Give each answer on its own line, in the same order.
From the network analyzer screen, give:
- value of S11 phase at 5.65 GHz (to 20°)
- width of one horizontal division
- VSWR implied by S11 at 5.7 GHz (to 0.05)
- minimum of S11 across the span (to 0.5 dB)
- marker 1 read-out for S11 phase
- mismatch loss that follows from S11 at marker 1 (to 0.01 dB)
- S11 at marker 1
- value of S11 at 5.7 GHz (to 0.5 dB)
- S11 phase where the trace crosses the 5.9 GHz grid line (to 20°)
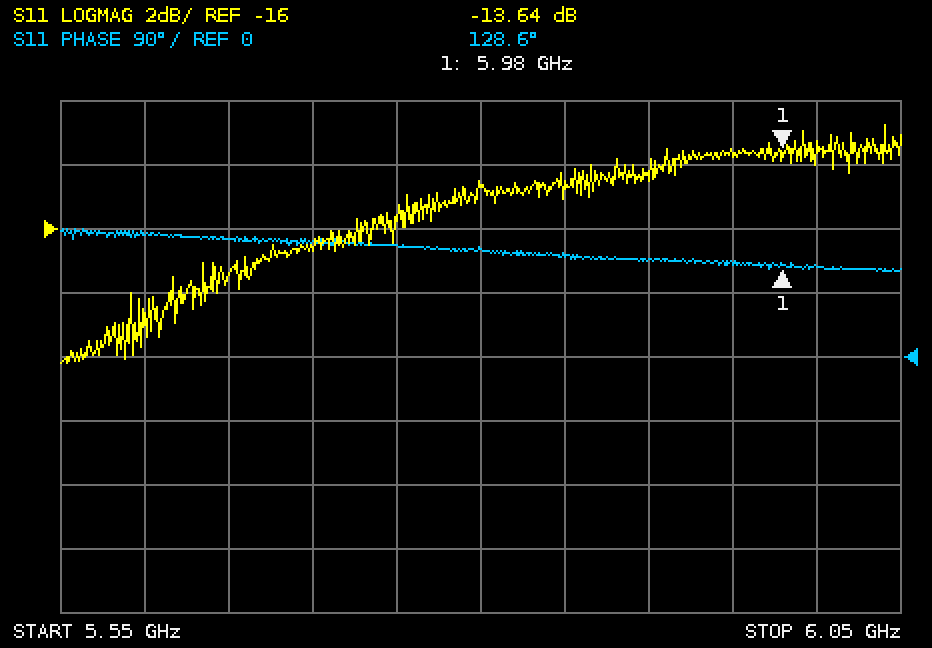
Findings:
160°
50 MHz
1.35
-20.0 dB
128.6°
0.19 dB
-13.64 dB
-16.5 dB
140°
